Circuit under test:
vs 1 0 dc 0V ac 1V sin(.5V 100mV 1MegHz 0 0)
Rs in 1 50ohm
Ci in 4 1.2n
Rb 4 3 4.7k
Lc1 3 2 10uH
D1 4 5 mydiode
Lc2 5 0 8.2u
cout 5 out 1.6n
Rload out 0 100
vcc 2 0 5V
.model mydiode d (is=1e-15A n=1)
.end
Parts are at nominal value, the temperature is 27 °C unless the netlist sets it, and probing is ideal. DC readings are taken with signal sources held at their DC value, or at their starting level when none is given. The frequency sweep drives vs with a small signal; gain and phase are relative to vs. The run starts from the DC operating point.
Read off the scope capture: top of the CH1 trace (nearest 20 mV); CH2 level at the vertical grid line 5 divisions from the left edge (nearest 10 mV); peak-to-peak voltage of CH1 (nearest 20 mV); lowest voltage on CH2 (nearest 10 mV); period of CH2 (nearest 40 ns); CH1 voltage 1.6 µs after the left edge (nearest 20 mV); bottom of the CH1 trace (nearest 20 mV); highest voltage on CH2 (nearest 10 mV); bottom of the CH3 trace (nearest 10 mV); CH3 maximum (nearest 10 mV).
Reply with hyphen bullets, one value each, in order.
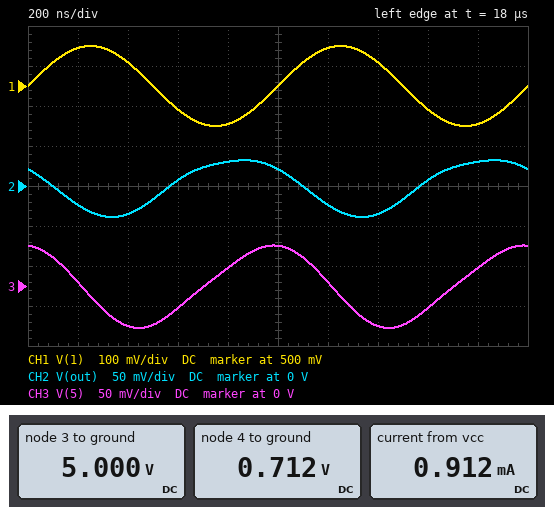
- 600 mV
- 20 mV
- 200 mV
- -40 mV
- 1.00 µs
- 440 mV
- 400 mV
- 30 mV
- -50 mV
- 50 mV
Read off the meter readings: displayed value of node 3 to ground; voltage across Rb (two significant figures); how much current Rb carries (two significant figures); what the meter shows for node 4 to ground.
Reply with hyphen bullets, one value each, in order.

- 5.000 V
- 4.3 V
- 910 µA
- 0.712 V
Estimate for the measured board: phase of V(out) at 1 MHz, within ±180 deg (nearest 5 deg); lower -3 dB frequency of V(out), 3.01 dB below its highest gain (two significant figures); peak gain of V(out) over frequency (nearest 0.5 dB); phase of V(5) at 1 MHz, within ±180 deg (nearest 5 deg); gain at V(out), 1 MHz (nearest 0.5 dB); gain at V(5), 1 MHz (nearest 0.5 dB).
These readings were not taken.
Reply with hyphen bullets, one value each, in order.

- 150 deg
- 1.0 MHz
- -5.0 dB
- 105 deg
- -8.5 dB
- -5.5 dB
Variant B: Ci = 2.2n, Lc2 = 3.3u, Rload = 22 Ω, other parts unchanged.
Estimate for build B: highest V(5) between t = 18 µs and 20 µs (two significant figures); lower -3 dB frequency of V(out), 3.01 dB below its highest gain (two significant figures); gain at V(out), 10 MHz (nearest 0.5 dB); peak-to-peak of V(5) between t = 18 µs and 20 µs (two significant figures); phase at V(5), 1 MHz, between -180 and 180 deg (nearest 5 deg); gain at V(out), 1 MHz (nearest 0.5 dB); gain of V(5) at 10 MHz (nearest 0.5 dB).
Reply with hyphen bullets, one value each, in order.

- 24 mV
- 1.5 MHz
- -13.0 dB
- 56 mV
- 115 deg
- -24.5 dB
- -12.5 dB
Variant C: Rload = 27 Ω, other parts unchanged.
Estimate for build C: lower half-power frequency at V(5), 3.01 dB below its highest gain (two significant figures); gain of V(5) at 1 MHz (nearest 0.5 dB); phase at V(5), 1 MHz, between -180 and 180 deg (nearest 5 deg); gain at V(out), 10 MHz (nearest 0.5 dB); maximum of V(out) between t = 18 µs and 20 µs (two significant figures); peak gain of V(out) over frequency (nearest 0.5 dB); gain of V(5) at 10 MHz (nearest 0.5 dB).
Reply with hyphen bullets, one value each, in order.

- 920 kHz
- -1.5 dB
- 95 deg
- -12.0 dB
- 21 mV
- -11.0 dB
- -11.5 dB
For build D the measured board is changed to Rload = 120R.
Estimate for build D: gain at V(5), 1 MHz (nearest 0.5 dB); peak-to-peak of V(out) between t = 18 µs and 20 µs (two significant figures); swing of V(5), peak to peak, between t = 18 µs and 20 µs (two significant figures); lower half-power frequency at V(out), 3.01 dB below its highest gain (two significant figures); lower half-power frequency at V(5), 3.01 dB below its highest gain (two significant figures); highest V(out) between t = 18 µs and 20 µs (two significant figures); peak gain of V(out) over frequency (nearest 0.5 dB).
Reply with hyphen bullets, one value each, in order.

- -6.0 dB
- 74 mV
- 99 mV
- 1.1 MHz
- 970 kHz
- 34 mV
- -4.5 dB
